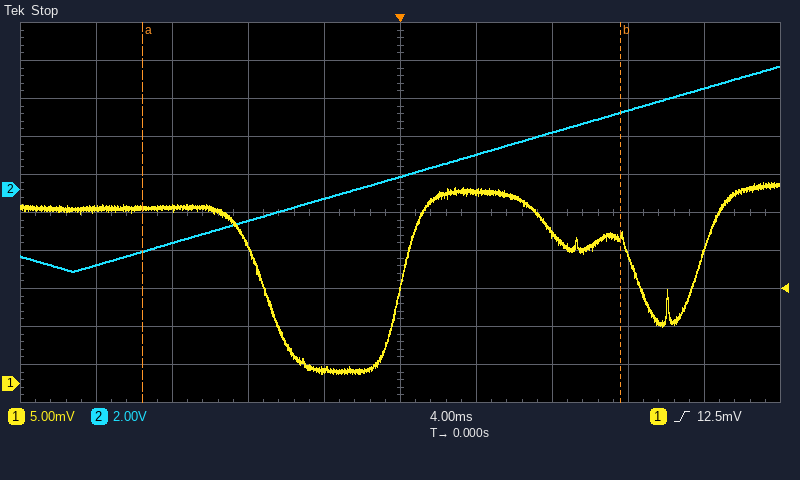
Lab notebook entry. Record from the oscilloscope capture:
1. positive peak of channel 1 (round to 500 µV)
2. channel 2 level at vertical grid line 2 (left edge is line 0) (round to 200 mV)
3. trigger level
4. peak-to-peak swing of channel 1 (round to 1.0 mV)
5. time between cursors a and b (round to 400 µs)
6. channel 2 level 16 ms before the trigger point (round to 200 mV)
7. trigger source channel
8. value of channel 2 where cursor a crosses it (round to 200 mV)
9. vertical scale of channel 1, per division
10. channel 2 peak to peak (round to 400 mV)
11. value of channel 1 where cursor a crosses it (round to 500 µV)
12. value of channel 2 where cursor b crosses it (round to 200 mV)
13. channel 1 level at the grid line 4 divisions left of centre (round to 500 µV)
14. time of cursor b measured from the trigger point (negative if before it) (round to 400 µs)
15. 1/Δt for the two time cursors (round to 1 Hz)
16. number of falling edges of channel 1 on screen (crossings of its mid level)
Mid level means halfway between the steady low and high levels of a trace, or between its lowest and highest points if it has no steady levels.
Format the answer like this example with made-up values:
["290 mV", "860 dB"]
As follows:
["26.5 mV", "-2.8 V", "12.5 mV", "25.0 mV", "25.2 ms", "-4.0 V", "channel 1", "-3.2 V", "5 mV", "10.8 V", "23.0 mV", "4.0 V", "23.0 mV", "+11.6 ms", "40 Hz", "2"]
